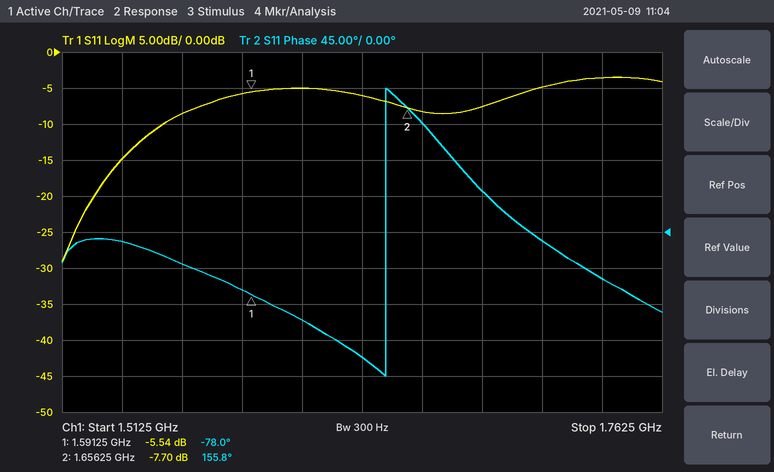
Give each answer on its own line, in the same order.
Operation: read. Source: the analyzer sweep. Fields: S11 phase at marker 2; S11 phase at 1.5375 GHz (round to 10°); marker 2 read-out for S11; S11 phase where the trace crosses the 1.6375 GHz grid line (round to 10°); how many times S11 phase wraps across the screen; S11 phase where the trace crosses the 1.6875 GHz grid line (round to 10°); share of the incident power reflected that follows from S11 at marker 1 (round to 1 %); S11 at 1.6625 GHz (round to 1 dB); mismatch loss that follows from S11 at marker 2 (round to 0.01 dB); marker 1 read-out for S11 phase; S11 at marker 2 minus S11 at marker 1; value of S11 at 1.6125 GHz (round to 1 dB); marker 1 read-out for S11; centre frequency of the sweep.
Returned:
155.8°
-10°
-7.70 dB
-160°
1
50°
28 %
-8 dB
0.81 dB
-78.0°
-2.16 dB
-5 dB
-5.54 dB
1.6375 GHz
